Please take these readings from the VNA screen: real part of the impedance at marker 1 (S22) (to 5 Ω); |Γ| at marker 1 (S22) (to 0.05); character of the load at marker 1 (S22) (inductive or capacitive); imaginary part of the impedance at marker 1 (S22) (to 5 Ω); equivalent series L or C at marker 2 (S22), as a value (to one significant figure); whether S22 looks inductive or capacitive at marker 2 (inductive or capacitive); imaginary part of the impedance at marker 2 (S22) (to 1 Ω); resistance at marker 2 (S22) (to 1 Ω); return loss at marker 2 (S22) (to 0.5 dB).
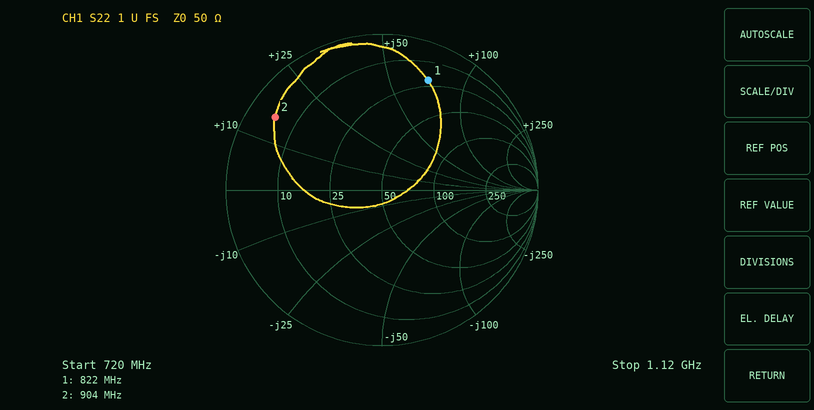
20 Ω
0.75
inductive
+70 Ω
3 nH
inductive
+15 Ω
5 Ω
1.5 dB
